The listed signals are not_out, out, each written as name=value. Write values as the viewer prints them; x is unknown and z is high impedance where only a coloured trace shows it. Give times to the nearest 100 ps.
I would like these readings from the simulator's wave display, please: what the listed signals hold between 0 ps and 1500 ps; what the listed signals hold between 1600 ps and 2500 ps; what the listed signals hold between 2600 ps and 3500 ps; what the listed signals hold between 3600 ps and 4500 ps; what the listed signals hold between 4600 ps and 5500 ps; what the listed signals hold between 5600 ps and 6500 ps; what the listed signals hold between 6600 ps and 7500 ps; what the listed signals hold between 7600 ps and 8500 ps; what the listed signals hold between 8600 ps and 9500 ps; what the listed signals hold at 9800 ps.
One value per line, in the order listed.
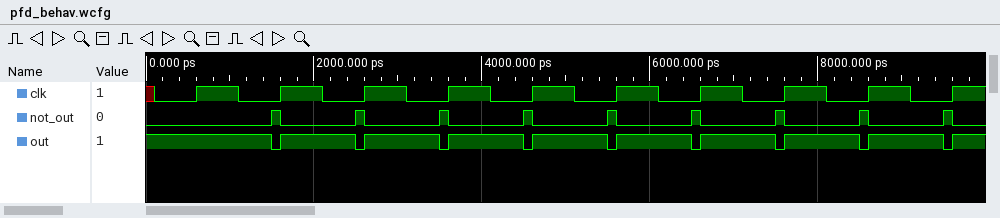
not_out=0, out=1
not_out=0, out=1
not_out=0, out=1
not_out=0, out=1
not_out=0, out=1
not_out=0, out=1
not_out=0, out=1
not_out=0, out=1
not_out=0, out=1
not_out=0, out=1
